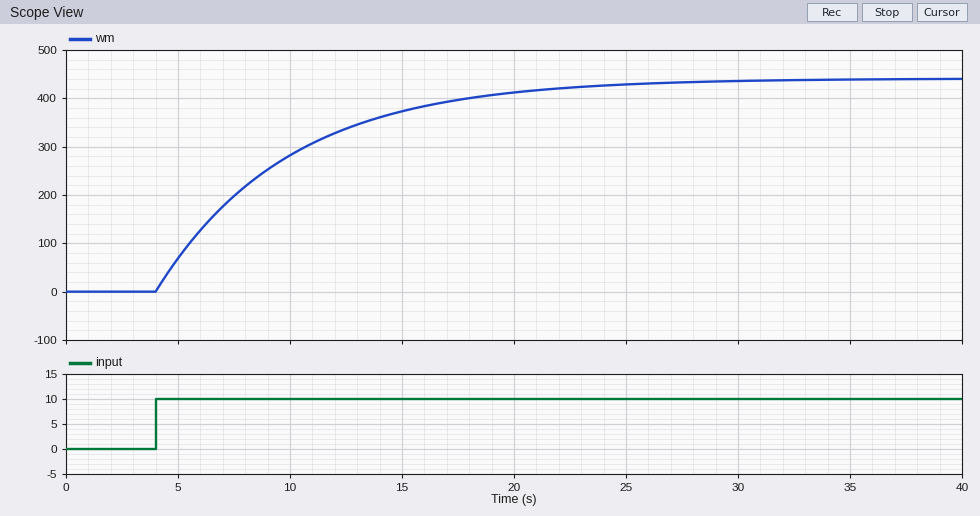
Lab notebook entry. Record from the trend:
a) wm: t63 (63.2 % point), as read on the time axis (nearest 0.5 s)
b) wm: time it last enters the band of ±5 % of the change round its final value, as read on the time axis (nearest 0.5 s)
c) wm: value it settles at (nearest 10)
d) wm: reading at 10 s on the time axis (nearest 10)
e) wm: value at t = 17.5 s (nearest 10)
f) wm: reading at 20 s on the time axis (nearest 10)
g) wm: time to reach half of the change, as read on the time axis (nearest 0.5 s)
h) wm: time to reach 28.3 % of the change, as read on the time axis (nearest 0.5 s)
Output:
10.0 s
21.5 s
440
280
400
410
8.0 s
6.0 s
